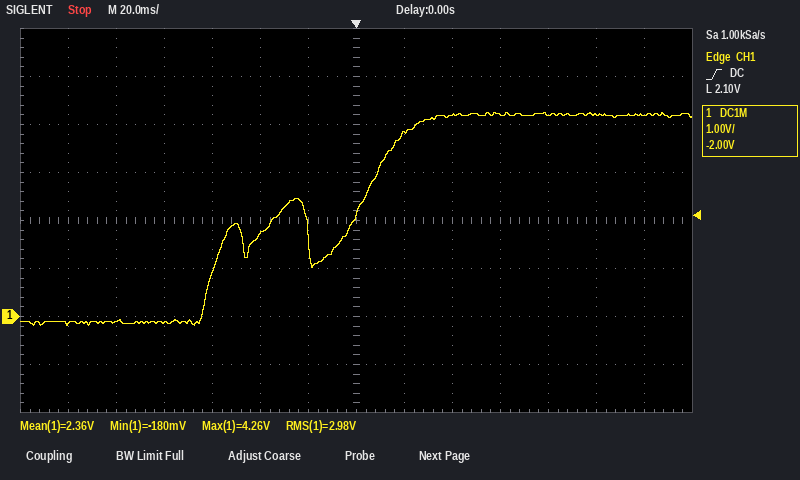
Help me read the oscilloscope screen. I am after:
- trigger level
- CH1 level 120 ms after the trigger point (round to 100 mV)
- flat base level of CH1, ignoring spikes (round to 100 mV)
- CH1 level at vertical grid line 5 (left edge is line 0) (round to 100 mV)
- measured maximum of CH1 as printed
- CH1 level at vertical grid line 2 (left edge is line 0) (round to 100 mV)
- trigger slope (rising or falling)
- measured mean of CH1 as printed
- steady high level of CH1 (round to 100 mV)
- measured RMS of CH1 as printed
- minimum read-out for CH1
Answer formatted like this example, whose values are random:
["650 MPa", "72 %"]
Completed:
["2.10 V", "4.2 V", "-100 mV", "1.7 V", "4.26 V", "-100 mV", "rising", "2.36 V", "4.2 V", "2.98 V", "-180 mV"]
